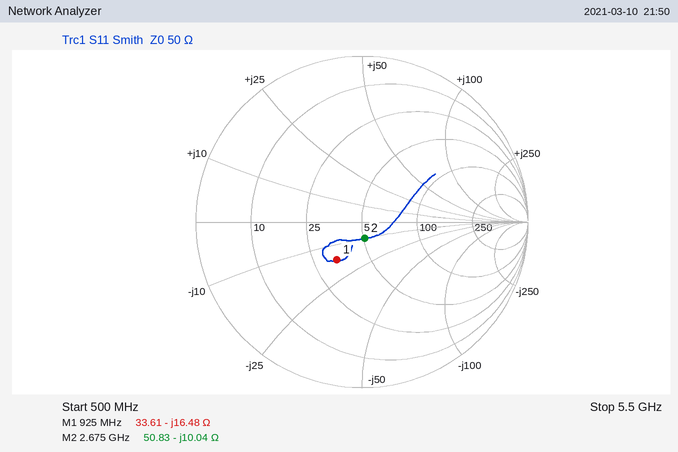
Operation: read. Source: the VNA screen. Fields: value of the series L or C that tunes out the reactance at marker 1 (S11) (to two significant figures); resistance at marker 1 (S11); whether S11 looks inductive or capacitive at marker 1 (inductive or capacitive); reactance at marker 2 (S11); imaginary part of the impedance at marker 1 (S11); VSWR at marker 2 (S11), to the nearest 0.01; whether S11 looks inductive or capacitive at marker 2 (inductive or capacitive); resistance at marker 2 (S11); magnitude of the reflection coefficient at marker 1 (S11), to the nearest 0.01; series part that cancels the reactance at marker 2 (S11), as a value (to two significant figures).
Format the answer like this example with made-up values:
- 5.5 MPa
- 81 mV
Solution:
- 2.8 nH
- 33.61 Ω
- capacitive
- -10.04 Ω
- -16.48 Ω
- 1.22
- capacitive
- 50.83 Ω
- 0.27
- 600 pH
